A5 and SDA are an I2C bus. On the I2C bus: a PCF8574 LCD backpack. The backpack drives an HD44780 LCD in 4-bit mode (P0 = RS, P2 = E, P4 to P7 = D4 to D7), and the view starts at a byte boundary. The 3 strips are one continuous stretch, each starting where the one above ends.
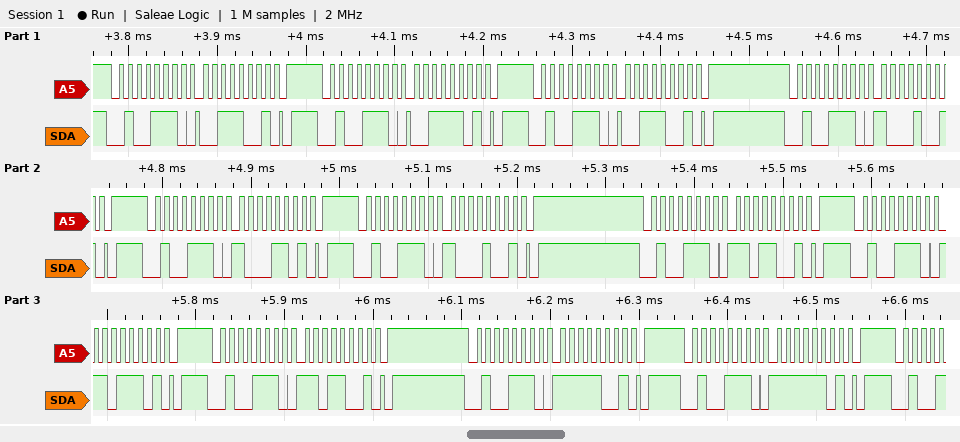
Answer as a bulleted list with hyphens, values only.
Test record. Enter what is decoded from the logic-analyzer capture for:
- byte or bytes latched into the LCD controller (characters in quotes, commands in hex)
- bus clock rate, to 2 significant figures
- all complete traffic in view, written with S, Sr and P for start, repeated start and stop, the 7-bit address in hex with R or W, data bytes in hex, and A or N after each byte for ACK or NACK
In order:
- '8'
- 100 kHz
- S 27W A 39 A P S 27W A 3D A P S 27W A 39 A P S 27W A 89 A P S 27W A 8D A P S 27W A 89 A P S 27W A D9 A P S 27W A DD A P S 27W A D9 A P S 27W A F9 A P S 27W A FD A P
